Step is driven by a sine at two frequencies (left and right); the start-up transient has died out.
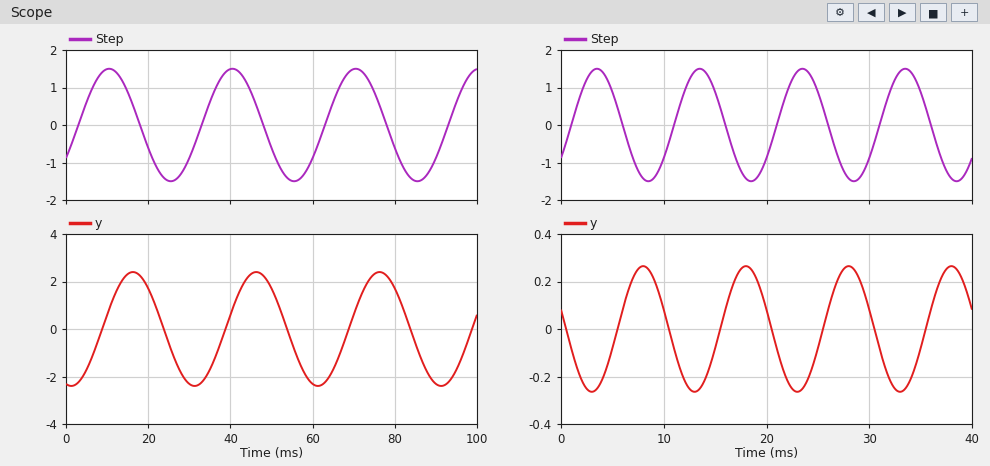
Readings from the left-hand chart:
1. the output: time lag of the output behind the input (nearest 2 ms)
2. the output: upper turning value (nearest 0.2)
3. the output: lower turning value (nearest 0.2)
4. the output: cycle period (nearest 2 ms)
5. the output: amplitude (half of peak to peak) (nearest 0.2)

6 ms
2.4
-2.4
30 ms
2.4
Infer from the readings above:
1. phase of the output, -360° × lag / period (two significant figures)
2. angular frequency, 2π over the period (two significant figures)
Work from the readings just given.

-72°
0.21 rad/ms
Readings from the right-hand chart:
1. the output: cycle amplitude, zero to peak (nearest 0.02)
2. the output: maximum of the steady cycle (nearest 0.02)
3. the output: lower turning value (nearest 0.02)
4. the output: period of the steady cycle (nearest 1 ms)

0.26
0.26
-0.26
10 ms
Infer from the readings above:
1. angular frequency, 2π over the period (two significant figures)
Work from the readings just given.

0.63 rad/ms
